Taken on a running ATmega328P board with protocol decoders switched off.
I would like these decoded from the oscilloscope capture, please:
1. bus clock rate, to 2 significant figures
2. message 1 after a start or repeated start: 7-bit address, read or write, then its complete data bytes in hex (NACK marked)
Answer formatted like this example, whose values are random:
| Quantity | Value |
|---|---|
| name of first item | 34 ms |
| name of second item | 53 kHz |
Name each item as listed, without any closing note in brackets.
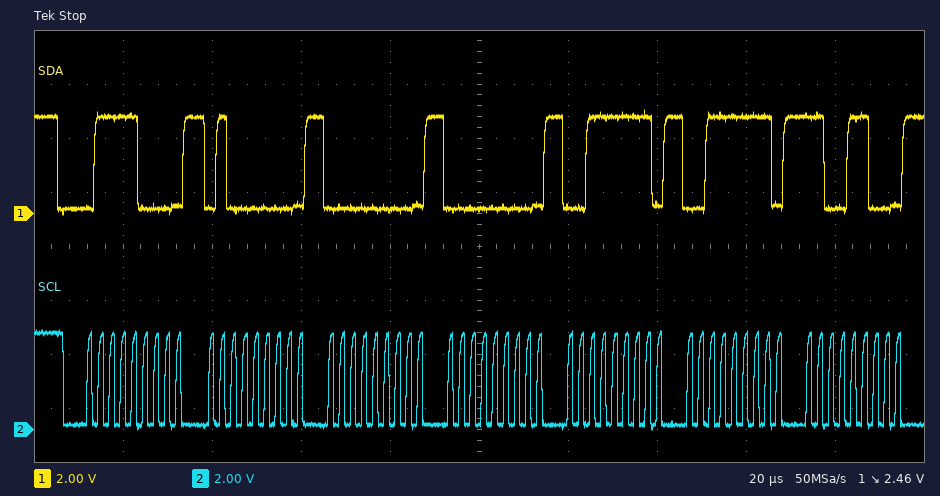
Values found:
| Quantity | Value |
|---|---|
| bus clock rate, to 2 significant figures | 400 kHz |
| message 1 after a start or repeated start: 7-bit address, read or write, then its complete data bytes in hex | 0x3C write: 40 00 00 3F 3F CC |
